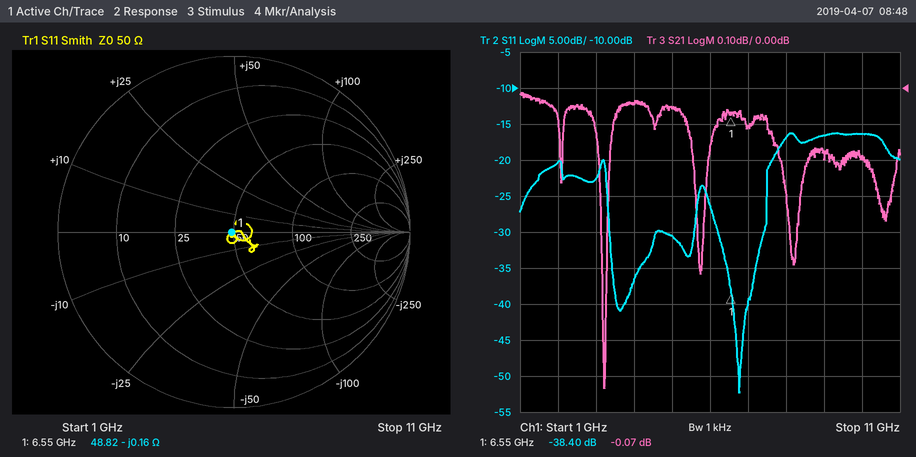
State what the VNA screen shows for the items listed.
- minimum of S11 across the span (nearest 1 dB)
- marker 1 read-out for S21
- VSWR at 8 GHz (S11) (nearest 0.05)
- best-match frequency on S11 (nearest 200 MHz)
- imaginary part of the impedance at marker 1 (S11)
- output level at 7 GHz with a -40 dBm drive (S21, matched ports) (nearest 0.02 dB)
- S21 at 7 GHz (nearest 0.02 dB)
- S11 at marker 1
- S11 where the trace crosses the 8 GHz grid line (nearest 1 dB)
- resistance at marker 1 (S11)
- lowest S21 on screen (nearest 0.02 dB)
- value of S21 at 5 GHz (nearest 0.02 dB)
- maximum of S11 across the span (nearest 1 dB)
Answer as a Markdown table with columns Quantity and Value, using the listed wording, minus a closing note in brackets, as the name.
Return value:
| Quantity | Value |
|---|---|
| minimum of S11 across the span | -52 dB |
| marker 1 read-out for S21 | -0.07 dB |
| VSWR at 8 GHz (S11) | 1.35 |
| best-match frequency on S11 | 6.8 GHz |
| imaginary part of the impedance at marker 1 | -0.16 Ω |
| output level at 7 GHz with a -40 dBm drive (S21, matched ports) | -40.10 dBm |
| S21 at 7 GHz | -0.10 dB |
| S11 at marker 1 | -38.40 dB |
| S11 where the trace crosses the 8 GHz grid line | -17 dB |
| resistance at marker 1 | 48.82 Ω |
| lowest S21 on screen | -0.84 dB |
| value of S21 at 5 GHz | -0.06 dB |
| maximum of S11 across the span | -16 dB |
